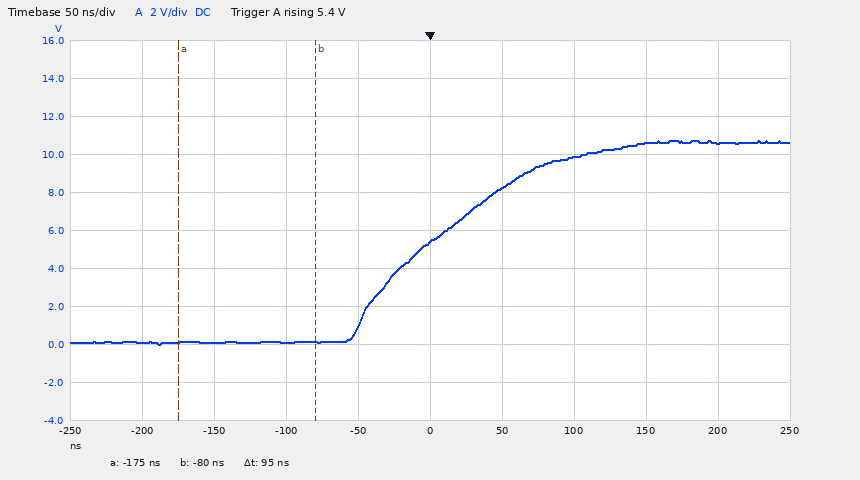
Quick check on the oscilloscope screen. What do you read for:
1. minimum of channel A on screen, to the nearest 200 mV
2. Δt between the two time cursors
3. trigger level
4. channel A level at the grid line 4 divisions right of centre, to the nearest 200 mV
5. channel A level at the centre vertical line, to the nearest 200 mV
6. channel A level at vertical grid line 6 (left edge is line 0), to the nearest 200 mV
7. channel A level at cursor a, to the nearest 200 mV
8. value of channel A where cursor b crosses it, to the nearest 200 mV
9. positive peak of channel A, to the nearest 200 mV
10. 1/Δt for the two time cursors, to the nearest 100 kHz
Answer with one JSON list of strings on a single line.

["0.0 V", "95 ns", "5.4 V", "10.6 V", "5.4 V", "8.2 V", "200 mV", "200 mV", "10.8 V", "10.5 MHz"]
